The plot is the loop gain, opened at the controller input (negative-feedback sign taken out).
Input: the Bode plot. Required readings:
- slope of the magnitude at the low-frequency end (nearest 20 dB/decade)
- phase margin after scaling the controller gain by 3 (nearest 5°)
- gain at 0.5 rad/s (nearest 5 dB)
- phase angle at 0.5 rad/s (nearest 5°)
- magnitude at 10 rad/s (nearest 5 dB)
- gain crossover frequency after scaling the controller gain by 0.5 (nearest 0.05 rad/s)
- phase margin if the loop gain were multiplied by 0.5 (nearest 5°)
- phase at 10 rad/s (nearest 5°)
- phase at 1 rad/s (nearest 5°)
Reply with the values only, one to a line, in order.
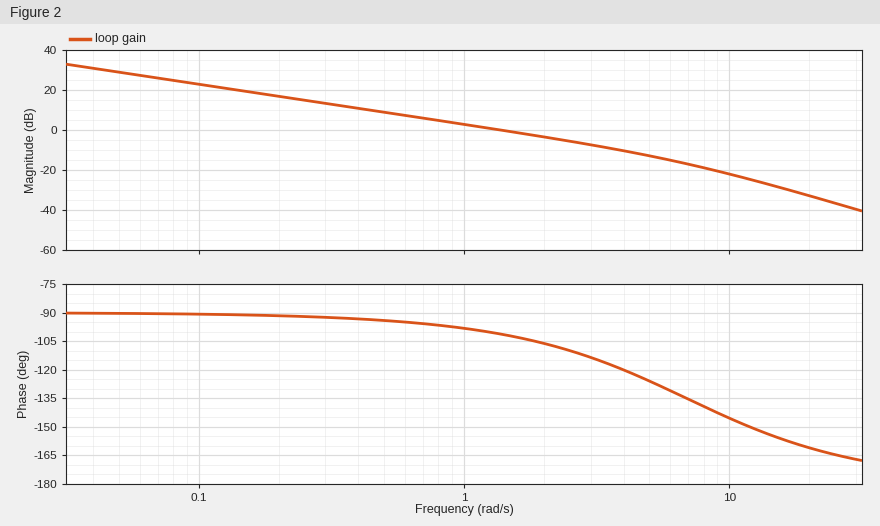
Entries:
-20 dB/decade
60°
10 dB
-95°
-20 dB
0.70 rad/s
85°
-145°
-100°
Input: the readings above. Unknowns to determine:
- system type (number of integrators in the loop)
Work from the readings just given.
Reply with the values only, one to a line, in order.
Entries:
1
